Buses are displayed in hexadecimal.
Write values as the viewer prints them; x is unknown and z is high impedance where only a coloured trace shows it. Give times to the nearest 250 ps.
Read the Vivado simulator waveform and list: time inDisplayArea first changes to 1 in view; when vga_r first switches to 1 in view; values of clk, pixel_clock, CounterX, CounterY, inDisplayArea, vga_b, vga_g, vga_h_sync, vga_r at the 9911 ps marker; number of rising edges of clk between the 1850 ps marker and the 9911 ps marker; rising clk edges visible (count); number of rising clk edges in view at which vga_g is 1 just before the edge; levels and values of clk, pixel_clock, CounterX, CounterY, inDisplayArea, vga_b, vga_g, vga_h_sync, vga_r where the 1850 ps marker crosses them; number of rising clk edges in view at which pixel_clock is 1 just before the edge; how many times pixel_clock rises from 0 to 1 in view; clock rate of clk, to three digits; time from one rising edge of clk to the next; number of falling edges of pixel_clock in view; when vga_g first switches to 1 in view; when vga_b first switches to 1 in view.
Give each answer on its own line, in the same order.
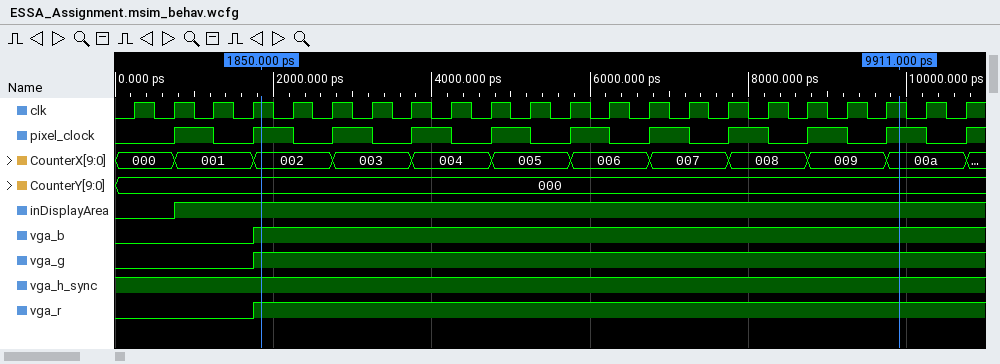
750 ps
1750 ps
clk=1, pixel_clock=1, CounterX=00a, CounterY=000, inDisplayArea=1, vga_b=1, vga_g=1, vga_h_sync=1, vga_r=1
16
22
18
clk=1, pixel_clock=1, CounterX=002, CounterY=000, inDisplayArea=1, vga_b=1, vga_g=1, vga_h_sync=1, vga_r=1
10
11
2.00 GHz
500 ps
10
1750 ps
1750 ps
